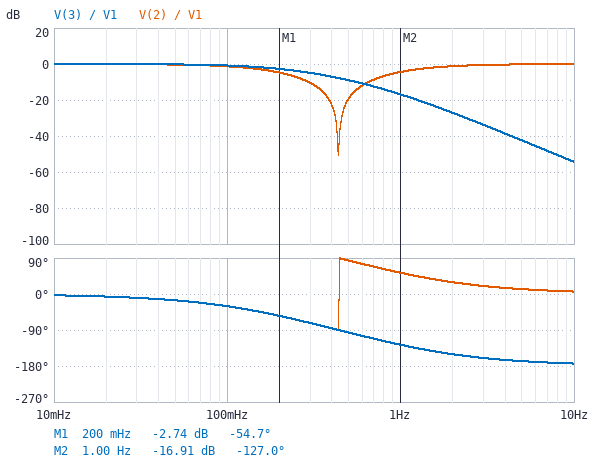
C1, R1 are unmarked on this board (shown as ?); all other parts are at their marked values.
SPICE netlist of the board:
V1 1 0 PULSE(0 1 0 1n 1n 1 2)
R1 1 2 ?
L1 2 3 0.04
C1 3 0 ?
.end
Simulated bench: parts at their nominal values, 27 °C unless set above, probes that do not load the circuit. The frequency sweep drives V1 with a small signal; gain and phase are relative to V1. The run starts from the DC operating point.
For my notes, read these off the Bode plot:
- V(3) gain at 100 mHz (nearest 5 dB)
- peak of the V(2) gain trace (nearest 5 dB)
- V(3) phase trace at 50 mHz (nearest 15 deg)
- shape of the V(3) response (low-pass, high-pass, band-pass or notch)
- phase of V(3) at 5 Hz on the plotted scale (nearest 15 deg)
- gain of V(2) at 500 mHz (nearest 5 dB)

0 dB
0 dB
-15 deg
low-pass
-165 deg
-20 dB
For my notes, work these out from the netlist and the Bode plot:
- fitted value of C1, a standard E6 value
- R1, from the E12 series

3.3 F
0.27 Ω
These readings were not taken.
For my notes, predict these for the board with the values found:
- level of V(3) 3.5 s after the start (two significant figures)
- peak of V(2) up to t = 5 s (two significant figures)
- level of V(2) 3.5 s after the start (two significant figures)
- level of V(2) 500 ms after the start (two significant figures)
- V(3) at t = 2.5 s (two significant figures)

510 mV
1.3 V
560 mV
270 mV
480 mV
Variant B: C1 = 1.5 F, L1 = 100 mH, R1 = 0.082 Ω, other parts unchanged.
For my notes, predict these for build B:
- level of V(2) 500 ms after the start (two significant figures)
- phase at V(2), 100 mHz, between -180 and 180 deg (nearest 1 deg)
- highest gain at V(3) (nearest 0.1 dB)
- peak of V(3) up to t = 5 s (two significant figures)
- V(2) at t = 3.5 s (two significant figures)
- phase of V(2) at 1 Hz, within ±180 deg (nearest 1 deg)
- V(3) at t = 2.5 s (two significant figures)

750 mV
-5 deg
10.1 dB
1.8 V
330 mV
9 deg
-200 mV
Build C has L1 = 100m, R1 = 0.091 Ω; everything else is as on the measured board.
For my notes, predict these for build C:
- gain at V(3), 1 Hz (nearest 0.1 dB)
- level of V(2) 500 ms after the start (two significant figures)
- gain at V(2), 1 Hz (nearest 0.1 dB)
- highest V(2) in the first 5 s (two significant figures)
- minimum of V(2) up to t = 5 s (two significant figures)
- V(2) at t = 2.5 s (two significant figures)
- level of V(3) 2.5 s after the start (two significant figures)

-21.7 dB
680 mV
-0.1 dB
1.4 V
-340 mV
990 mV
210 mV
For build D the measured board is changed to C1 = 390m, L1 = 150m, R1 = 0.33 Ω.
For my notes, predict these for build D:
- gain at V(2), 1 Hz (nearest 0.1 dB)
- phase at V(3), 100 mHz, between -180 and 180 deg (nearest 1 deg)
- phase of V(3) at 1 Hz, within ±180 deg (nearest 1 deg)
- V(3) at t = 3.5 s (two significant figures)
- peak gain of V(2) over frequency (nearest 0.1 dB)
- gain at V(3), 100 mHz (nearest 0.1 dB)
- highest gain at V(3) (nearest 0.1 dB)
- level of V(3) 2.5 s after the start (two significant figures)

-1.4 dB
-5 deg
-148 deg
-330 mV
0 dB
0.2 dB
5.8 dB
1.3 V
